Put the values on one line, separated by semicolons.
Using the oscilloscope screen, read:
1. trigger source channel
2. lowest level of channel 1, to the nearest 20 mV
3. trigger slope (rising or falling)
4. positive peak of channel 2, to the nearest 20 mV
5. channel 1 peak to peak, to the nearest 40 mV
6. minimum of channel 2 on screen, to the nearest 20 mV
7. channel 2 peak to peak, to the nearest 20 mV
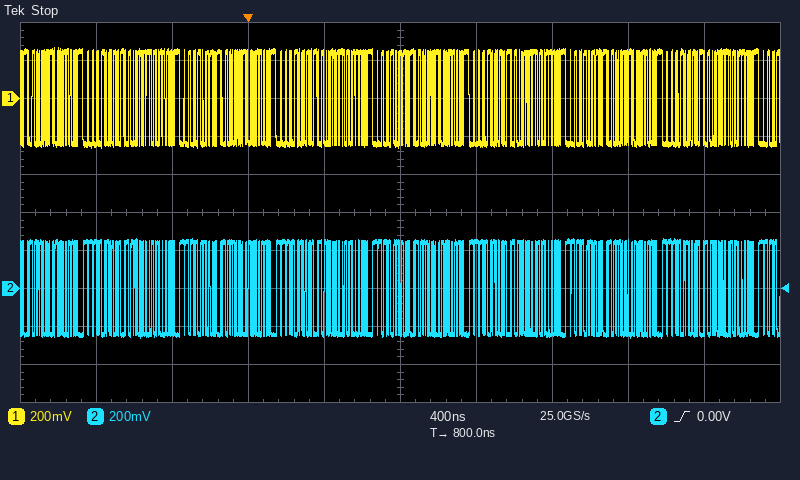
channel 2; -260 mV; rising; 260 mV; 520 mV; -260 mV; 520 mV
